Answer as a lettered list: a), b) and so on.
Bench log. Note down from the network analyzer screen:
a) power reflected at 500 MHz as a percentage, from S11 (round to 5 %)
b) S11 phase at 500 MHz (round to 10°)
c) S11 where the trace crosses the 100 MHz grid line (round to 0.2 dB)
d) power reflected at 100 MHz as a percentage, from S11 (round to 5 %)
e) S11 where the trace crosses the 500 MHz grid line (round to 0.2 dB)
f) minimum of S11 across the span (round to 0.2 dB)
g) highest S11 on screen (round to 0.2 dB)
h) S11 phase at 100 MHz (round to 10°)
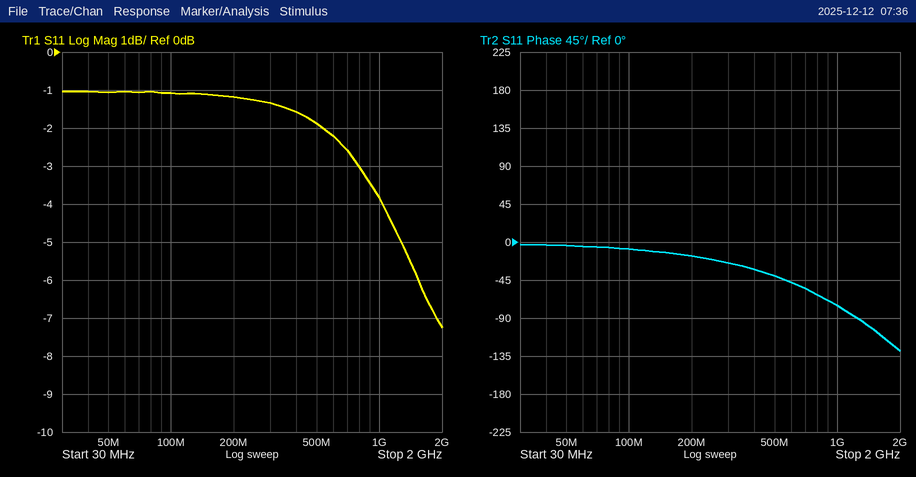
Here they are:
a) 65 %
b) -40°
c) -1.0 dB
d) 80 %
e) -1.8 dB
f) -7.2 dB
g) -1.0 dB
h) -10°
